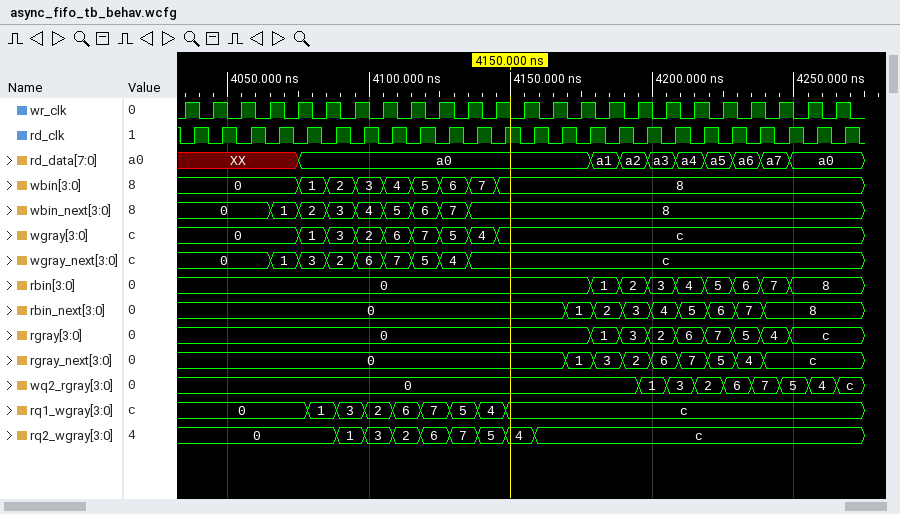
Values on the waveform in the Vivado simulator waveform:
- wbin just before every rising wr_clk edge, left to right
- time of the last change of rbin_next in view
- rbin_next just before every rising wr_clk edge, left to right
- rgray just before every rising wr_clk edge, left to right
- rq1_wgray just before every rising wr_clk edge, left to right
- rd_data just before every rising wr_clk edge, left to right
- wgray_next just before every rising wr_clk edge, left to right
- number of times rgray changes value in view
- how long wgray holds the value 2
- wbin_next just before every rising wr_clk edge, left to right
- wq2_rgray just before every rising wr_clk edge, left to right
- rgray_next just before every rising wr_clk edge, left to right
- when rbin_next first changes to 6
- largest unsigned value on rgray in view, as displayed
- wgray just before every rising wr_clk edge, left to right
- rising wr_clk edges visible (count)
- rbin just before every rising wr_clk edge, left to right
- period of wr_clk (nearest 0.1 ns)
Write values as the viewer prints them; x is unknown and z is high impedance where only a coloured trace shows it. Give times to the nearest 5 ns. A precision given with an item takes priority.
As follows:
0, 0, 0, 0, 0, 1, 2, 3, 4, 5, 6, 7, 8, 8, 8, 8, 8, 8, 8, 8, 8, 8, 8, 8
4240 ns
0, 0, 0, 0, 0, 0, 0, 0, 0, 0, 0, 0, 0, 0, 1, 2, 3, 4, 5, 6, 7, 8, 8, 8
0, 0, 0, 0, 0, 0, 0, 0, 0, 0, 0, 0, 0, 0, 0, 1, 3, 2, 6, 7, 5, 4, c, c
0, 0, 0, 0, 0, 1, 3, 2, 6, 7, 5, 4, c, c, c, c, c, c, c, c, c, c, c, c
XX, XX, XX, XX, XX, a0, a0, a0, a0, a0, a0, a0, a0, a0, a0, a1, a2, a3, a4, a5, a6, a7, a0, a0
0, 0, 0, 0, 1, 3, 2, 6, 7, 5, 4, c, c, c, c, c, c, c, c, c, c, c, c, c
8
10 ns
0, 0, 0, 0, 1, 2, 3, 4, 5, 6, 7, 8, 8, 8, 8, 8, 8, 8, 8, 8, 8, 8, 8, 8
0, 0, 0, 0, 0, 0, 0, 0, 0, 0, 0, 0, 0, 0, 0, 0, 0, 1, 3, 2, 6, 7, 5, 4
0, 0, 0, 0, 0, 0, 0, 0, 0, 0, 0, 0, 0, 0, 1, 3, 2, 6, 7, 5, 4, c, c, c
4220 ns
c
0, 0, 0, 0, 0, 1, 3, 2, 6, 7, 5, 4, c, c, c, c, c, c, c, c, c, c, c, c
24
0, 0, 0, 0, 0, 0, 0, 0, 0, 0, 0, 0, 0, 0, 0, 1, 2, 3, 4, 5, 6, 7, 8, 8
10 ns
